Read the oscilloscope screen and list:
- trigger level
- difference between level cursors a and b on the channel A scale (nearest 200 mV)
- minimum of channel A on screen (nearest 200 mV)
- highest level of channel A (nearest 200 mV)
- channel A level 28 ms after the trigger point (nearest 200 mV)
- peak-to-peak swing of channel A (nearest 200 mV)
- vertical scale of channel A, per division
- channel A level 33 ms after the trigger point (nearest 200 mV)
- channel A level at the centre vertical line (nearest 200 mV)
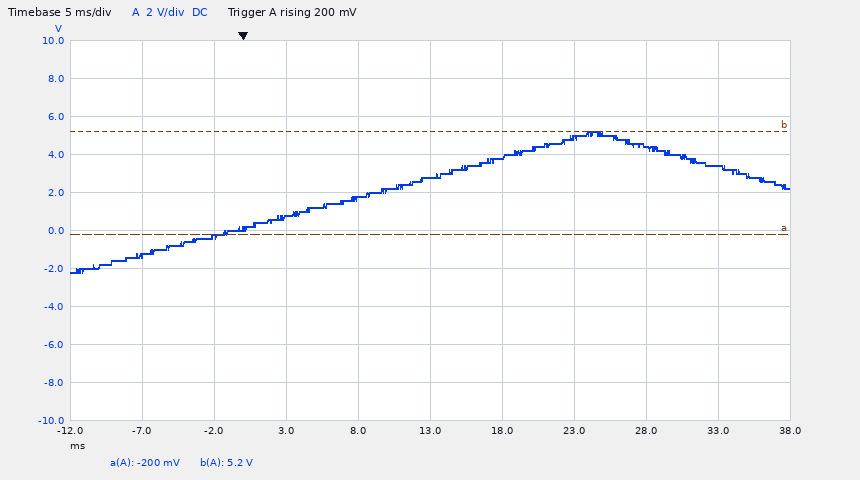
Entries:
200 mV
5.4 V
-2.2 V
5.2 V
4.4 V
7.4 V
2 V
3.4 V
2.8 V
